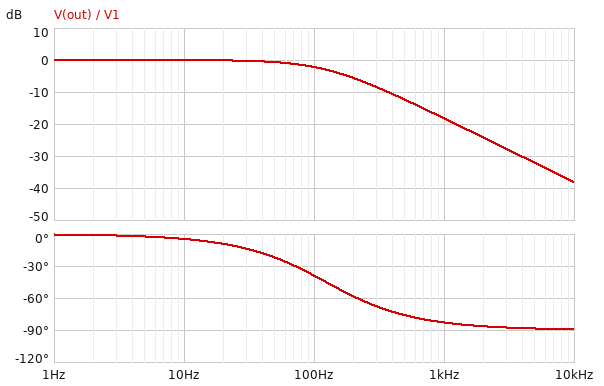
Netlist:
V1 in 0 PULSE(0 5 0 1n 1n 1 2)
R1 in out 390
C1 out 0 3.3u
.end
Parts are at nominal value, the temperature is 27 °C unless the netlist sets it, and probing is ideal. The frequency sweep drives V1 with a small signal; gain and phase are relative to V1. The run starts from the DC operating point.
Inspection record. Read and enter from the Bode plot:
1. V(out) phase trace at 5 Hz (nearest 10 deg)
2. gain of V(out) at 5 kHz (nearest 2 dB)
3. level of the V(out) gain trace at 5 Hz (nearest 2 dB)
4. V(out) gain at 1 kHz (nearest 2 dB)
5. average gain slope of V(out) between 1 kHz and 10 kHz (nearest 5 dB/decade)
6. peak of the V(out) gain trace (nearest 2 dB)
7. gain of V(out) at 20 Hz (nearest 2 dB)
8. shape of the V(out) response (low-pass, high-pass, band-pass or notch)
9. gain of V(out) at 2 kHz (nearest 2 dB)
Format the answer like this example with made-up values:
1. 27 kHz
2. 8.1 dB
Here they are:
1. 0 deg
2. -32 dB
3. 0 dB
4. -18 dB
5. -20 dB/decade
6. 0 dB
7. 0 dB
8. low-pass
9. -24 dB
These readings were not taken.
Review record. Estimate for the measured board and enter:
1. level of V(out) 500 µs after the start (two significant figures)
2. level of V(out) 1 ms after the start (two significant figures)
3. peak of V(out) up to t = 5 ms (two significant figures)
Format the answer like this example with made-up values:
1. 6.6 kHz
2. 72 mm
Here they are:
1. 1.6 V
2. 2.7 V
3. 4.9 V
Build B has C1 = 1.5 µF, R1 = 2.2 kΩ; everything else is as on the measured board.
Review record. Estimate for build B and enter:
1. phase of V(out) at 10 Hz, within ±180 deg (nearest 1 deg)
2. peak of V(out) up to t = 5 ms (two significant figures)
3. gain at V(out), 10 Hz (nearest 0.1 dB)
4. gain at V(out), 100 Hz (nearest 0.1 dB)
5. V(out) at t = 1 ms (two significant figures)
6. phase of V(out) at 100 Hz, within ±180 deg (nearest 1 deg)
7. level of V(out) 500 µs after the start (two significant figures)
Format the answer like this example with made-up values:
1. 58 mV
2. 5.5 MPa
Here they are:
1. -12 deg
2. 3.9 V
3. -0.2 dB
4. -7.2 dB
5. 1.3 V
6. -64 deg
7. 700 mV
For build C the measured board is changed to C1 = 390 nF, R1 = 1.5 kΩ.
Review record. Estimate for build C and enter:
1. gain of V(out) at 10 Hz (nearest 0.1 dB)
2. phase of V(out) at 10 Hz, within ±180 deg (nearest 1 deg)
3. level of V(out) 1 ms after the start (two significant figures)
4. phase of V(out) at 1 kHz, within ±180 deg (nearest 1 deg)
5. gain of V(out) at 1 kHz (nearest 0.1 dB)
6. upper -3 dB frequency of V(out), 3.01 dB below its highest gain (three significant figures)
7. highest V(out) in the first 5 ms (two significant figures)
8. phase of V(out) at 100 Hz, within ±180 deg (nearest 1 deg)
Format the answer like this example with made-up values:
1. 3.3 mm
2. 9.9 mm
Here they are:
1. 0 dB
2. -2 deg
3. 4.1 V
4. -75 deg
5. -11.6 dB
6. 272 Hz
7. 5.0 V
8. -20 deg
